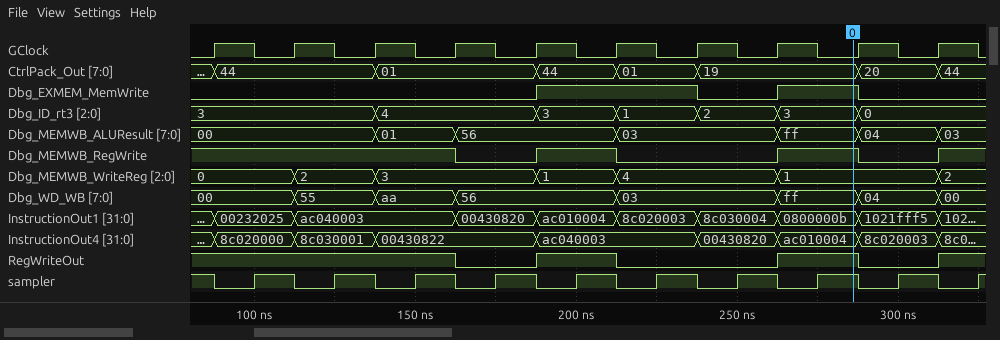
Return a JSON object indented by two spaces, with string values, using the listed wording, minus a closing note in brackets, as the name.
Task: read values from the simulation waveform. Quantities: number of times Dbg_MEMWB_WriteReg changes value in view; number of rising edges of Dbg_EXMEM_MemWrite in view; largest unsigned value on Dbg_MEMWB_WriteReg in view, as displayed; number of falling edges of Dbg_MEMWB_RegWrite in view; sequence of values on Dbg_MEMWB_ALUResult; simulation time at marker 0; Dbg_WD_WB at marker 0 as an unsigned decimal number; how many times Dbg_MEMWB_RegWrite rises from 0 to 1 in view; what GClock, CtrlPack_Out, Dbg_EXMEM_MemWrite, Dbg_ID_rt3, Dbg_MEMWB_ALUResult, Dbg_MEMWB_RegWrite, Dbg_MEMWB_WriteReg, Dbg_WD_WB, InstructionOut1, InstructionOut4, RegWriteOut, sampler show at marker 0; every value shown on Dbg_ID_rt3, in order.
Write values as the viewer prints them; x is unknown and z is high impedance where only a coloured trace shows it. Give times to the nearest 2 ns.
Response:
{
  "number of times Dbg_MEMWB_WriteReg changes value in view": "6",
  "number of rising edges of Dbg_EXMEM_MemWrite in view": "2",
  "largest unsigned value on Dbg_MEMWB_WriteReg in view, as displayed": "4",
  "number of falling edges of Dbg_MEMWB_RegWrite in view": "3",
  "sequence of values on Dbg_MEMWB_ALUResult": "00, 01, 56, 03, ff, 04, 03",
  "simulation time at marker 0": "286 ns",
  "Dbg_WD_WB at marker 0 as an unsigned decimal number": "255",
  "how many times Dbg_MEMWB_RegWrite rises from 0 to 1 in view": "3",
  "what GClock, CtrlPack_Out, Dbg_EXMEM_MemWrite, Dbg_ID_rt3, Dbg_MEMWB_ALUResult, Dbg_MEMWB_RegWrite, Dbg_MEMWB_WriteReg, Dbg_WD_WB, InstructionOut1, InstructionOut4, RegWriteOut, sampler show at marker 0": "GClock=0, CtrlPack_Out=19, Dbg_EXMEM_MemWrite=1, Dbg_ID_rt3=3, Dbg_MEMWB_ALUResult=ff, Dbg_MEMWB_RegWrite=1, Dbg_MEMWB_WriteReg=1, Dbg_WD_WB=ff, InstructionOut1=0800000b, InstructionOut4=ac010004, RegWriteOut=1, sampler=1",
  "every value shown on Dbg_ID_rt3, in order": "3, 4, 3, 1, 2, 3, 0"
}
